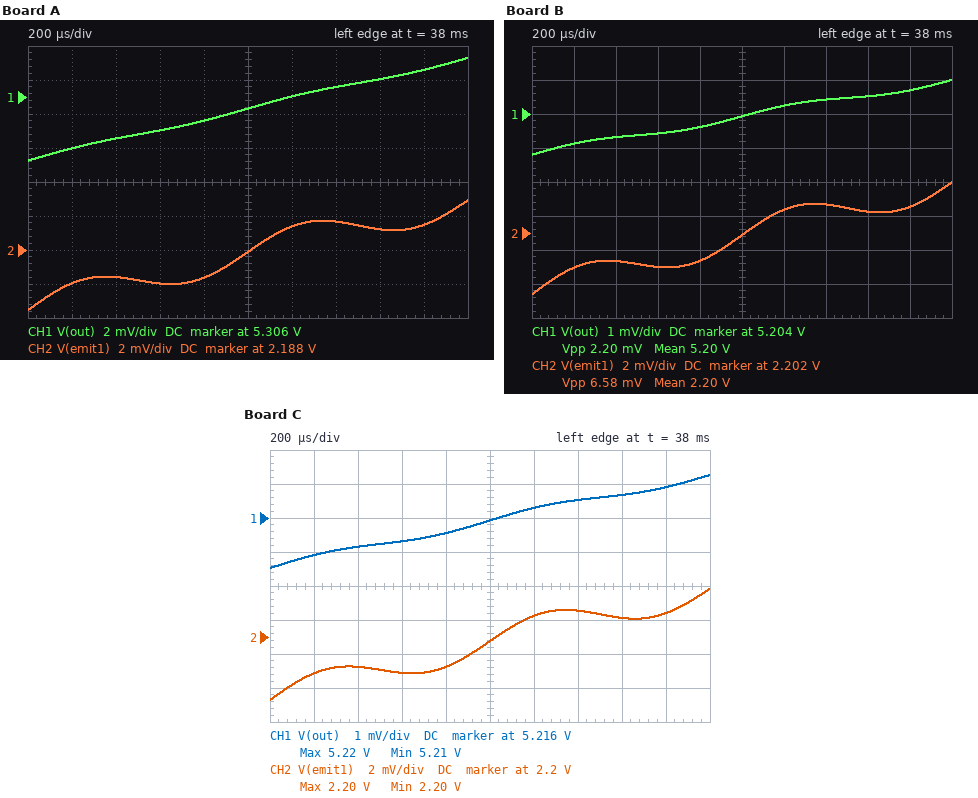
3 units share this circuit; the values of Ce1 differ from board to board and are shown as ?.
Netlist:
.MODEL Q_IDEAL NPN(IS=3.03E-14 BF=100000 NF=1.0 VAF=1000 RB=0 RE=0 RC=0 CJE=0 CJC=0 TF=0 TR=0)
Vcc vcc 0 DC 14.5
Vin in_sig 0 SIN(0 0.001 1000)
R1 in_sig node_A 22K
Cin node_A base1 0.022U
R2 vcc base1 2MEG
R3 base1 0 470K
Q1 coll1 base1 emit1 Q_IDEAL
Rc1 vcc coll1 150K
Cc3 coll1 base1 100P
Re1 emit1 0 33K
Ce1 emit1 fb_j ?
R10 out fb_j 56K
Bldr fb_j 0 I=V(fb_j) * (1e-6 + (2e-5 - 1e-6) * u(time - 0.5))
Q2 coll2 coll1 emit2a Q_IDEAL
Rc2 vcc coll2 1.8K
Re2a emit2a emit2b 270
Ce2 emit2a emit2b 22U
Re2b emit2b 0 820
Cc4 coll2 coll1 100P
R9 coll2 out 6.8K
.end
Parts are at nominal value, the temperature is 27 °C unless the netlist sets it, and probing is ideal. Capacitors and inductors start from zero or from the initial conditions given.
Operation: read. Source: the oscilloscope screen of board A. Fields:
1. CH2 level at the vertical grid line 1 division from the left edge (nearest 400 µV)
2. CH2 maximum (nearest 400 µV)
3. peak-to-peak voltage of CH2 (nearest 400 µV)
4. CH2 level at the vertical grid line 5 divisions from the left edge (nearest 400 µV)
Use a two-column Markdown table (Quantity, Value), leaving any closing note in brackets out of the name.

| Quantity | Value |
|---|---|
| CH2 level at the vertical grid line 1 division from the left edge | 2.1860 V |
| CH2 maximum | 2.1908 V |
| peak-to-peak voltage of CH2 | 6.4 mV |
| CH2 level at the vertical grid line 5 divisions from the left edge | 2.1880 V |
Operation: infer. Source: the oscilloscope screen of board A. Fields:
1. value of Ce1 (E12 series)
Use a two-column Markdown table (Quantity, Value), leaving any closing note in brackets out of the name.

| Quantity | Value |
|---|---|
| value of Ce1 | 1.5 µF |
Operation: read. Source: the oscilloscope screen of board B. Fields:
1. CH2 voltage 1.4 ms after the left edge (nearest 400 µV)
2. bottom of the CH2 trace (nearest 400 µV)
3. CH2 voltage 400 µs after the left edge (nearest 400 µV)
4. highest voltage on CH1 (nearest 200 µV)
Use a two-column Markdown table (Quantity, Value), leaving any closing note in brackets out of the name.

| Quantity | Value |
|---|---|
| CH2 voltage 1.4 ms after the left edge | 2.2036 V |
| bottom of the CH2 trace | 2.1984 V |
| CH2 voltage 400 µs after the left edge | 2.2004 V |
| highest voltage on CH1 | 5.2050 V |
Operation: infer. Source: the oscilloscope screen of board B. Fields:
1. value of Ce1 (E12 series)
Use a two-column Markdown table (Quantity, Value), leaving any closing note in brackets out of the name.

| Quantity | Value |
|---|---|
| value of Ce1 | 8.2 µF |
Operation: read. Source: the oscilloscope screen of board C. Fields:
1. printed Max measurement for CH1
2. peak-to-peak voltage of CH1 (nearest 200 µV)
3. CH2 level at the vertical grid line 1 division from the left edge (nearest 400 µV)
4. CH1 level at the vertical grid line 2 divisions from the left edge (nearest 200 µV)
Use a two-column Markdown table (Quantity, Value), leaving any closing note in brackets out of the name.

| Quantity | Value |
|---|---|
| printed Max measurement for CH1 | 5.22 V |
| peak-to-peak voltage of CH1 | 2.8 mV |
| CH2 level at the vertical grid line 1 division from the left edge | 2.1980 V |
| CH1 level at the vertical grid line 2 divisions from the left edge | 5.2152 V |
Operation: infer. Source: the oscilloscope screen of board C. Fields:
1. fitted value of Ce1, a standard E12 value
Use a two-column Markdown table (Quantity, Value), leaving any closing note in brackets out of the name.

| Quantity | Value |
|---|---|
| fitted value of Ce1, a standard E12 value | 5.6 µF |
